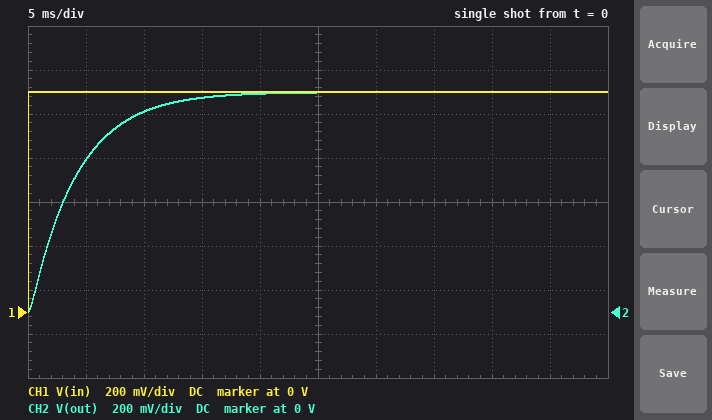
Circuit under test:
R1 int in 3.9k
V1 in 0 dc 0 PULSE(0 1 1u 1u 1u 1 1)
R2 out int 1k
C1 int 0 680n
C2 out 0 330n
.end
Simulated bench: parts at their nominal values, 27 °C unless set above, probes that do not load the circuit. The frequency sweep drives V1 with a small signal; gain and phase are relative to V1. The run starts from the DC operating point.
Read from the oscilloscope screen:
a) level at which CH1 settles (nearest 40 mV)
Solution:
1.00 V
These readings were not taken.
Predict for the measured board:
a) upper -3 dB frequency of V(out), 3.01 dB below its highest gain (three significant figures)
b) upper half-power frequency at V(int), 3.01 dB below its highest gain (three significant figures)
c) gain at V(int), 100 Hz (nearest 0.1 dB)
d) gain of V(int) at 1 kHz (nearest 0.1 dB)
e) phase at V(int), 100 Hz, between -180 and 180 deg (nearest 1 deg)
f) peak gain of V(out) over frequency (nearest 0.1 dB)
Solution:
39.2 Hz
39.4 Hz
-8.6 dB
-25.4 dB
-65 deg
0 dB
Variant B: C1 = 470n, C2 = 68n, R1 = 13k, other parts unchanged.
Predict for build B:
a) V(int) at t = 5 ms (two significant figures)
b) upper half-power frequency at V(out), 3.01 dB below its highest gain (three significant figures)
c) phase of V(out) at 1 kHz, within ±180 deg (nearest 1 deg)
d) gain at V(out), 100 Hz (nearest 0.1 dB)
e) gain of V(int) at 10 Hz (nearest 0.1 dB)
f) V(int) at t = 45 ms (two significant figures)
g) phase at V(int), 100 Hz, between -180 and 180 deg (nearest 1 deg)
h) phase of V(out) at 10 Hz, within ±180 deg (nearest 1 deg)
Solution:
510 mV
22.7 Hz
-109 deg
-13.1 dB
-0.8 dB
1.0 V
-77 deg
-24 deg
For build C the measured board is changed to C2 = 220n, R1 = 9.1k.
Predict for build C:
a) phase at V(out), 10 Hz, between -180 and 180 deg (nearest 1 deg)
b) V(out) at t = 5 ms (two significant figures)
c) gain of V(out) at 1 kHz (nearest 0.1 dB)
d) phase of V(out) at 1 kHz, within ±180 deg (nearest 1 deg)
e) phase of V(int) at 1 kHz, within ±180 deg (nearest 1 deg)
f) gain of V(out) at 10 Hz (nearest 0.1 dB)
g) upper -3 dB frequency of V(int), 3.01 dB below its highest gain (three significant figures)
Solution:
-28 deg
440 mV
-37.5 dB
-135 deg
-81 deg
-1.0 dB
19.3 Hz
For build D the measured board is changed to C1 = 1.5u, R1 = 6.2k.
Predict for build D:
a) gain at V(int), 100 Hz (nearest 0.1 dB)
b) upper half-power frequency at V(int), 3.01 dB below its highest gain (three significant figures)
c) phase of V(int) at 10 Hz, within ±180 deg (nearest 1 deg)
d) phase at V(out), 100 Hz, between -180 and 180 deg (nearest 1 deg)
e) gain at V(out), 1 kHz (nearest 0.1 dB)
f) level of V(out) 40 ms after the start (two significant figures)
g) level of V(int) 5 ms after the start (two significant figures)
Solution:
-17.1 dB
14.0 Hz
-35 deg
-92 deg
-43.0 dB
970 mV
360 mV
